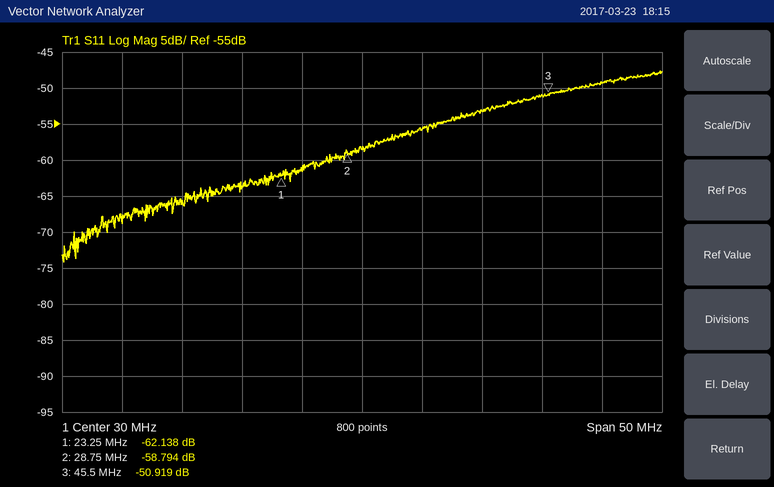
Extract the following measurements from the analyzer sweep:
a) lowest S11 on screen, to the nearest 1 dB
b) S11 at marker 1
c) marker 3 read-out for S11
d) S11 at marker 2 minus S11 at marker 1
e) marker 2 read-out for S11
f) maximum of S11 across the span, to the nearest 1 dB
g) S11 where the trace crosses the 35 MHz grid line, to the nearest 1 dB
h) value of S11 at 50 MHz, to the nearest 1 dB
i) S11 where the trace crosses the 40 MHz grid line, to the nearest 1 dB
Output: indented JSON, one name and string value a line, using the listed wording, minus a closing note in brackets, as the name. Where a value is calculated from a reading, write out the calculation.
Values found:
{
  "lowest S11 on screen, to the nearest 1 dB": "-74 dB",
  "S11 at marker 1": "-62.138 dB",
  "marker 3 read-out for S11": "-50.919 dB",
  "S11 at marker 2 minus S11 at marker 1": "-58.794 − (-62.138) = 3.344 dB",
  "marker 2 read-out for S11": "-58.794 dB",
  "maximum of S11 across the span, to the nearest 1 dB": "-48 dB",
  "S11 where the trace crosses the 35 MHz grid line, to the nearest 1 dB": "-56 dB",
  "value of S11 at 50 MHz, to the nearest 1 dB": "-49 dB",
  "S11 where the trace crosses the 40 MHz grid line, to the nearest 1 dB": "-53 dB"
}
